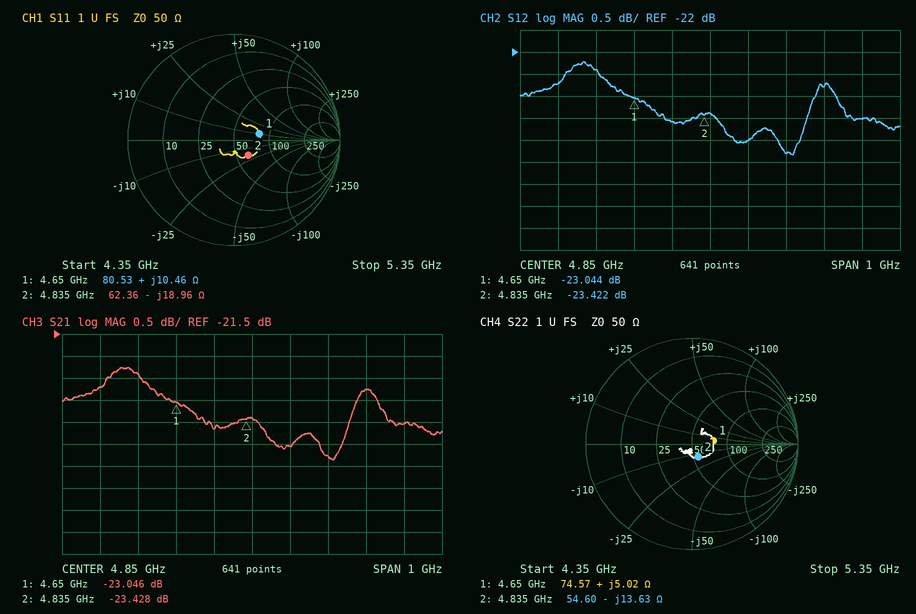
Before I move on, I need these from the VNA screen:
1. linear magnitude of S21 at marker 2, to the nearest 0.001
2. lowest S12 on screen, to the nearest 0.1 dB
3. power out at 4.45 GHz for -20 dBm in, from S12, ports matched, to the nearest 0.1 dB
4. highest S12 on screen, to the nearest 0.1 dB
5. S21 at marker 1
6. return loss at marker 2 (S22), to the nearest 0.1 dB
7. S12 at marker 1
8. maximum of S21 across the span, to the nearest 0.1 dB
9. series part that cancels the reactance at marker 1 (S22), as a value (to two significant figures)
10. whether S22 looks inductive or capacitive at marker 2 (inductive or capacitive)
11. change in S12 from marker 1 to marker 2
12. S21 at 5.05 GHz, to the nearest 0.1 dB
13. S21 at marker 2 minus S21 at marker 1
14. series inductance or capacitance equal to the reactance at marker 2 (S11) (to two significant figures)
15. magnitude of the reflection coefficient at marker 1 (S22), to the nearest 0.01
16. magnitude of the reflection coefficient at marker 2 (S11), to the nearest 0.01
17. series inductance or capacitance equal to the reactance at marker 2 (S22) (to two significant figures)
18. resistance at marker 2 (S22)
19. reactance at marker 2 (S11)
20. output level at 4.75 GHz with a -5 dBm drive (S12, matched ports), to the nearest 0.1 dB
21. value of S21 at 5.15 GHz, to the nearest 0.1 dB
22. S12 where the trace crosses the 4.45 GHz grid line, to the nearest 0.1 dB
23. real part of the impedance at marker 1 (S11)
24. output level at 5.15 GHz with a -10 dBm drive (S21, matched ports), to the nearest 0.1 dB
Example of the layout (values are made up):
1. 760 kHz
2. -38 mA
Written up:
1. 0.067
2. -24.3 dB
3. -42.7 dBm
4. -22.2 dB
5. -23.046 dB
6. 17.3 dB
7. -23.044 dB
8. -22.3 dB
9. 6.8 pF
10. capacitive
11. -0.378 dB
12. -24.3 dB
13. -0.382 dB
14. 1.7 pF
15. 0.20
16. 0.20
17. 2.4 pF
18. 54.60 Ω
19. -18.96 Ω
20. -28.6 dBm
21. -22.8 dB
22. -22.7 dB
23. 80.53 Ω
24. -32.8 dBm
